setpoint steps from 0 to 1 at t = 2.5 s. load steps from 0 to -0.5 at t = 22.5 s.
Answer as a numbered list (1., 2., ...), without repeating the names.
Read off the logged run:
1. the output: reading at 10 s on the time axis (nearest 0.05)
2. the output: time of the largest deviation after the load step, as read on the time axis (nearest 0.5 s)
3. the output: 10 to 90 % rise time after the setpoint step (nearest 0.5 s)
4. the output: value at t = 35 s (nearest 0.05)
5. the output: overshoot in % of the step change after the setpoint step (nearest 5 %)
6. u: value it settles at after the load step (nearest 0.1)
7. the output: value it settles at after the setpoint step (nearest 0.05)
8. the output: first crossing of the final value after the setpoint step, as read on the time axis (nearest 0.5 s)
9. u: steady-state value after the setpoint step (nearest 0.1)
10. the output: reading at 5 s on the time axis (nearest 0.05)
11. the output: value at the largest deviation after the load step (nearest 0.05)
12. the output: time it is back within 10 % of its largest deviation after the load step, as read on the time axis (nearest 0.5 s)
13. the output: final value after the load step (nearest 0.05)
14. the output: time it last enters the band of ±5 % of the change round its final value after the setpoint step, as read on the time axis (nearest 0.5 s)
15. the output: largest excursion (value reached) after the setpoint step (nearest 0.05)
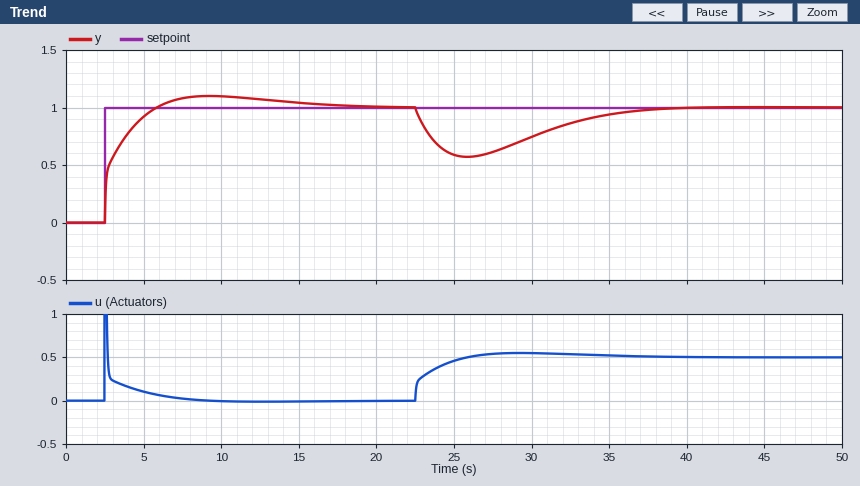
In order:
1. 1.10
2. 26.0 s
3. 2.5 s
4. 0.95
5. 10 %
6. 0.5
7. 1.00
8. 6.0 s
9. 0.0
10. 0.90
11. 0.55
12. 36.0 s
13. 1.00
14. 14.0 s
15. 1.10
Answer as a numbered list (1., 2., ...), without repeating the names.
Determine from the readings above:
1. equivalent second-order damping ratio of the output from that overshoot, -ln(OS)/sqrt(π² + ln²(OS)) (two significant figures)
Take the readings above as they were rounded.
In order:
1. 0.59
